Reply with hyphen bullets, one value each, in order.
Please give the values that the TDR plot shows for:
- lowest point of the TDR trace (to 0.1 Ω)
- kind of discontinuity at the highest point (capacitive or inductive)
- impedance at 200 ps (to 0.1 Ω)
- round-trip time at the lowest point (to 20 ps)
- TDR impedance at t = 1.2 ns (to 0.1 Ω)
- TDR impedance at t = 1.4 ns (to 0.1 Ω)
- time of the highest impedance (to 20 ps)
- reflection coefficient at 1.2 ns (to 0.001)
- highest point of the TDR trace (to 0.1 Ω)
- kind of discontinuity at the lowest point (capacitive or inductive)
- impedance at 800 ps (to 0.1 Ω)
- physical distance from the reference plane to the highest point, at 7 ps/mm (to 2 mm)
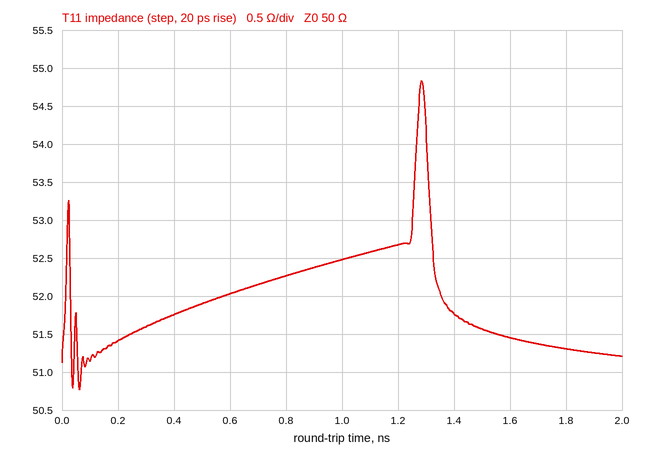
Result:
- 50.8 Ω
- inductive
- 51.4 Ω
- 60 ps
- 52.7 Ω
- 51.8 Ω
- 1.28 ns
- +0.026
- 54.8 Ω
- capacitive
- 52.3 Ω
- 92 mm
